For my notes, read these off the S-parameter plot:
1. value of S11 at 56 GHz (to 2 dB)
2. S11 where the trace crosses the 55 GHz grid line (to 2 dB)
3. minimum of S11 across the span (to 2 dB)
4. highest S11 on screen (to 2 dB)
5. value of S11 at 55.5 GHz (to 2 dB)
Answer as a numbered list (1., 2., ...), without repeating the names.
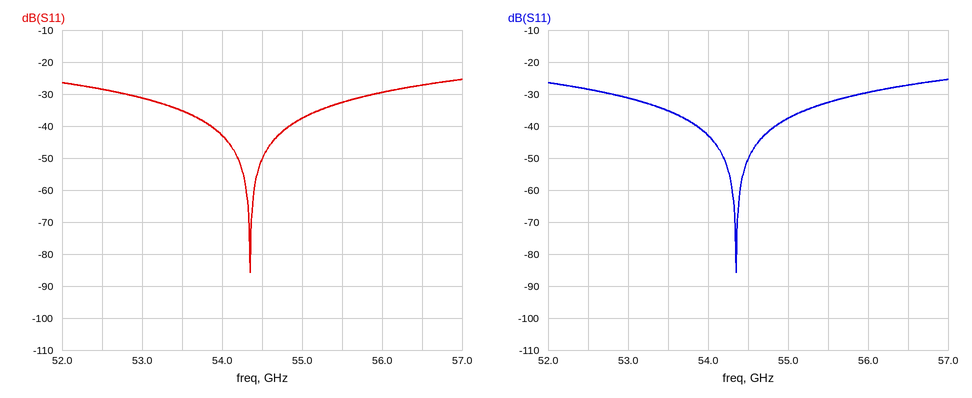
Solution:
1. -30 dB
2. -38 dB
3. -86 dB
4. -26 dB
5. -32 dB
